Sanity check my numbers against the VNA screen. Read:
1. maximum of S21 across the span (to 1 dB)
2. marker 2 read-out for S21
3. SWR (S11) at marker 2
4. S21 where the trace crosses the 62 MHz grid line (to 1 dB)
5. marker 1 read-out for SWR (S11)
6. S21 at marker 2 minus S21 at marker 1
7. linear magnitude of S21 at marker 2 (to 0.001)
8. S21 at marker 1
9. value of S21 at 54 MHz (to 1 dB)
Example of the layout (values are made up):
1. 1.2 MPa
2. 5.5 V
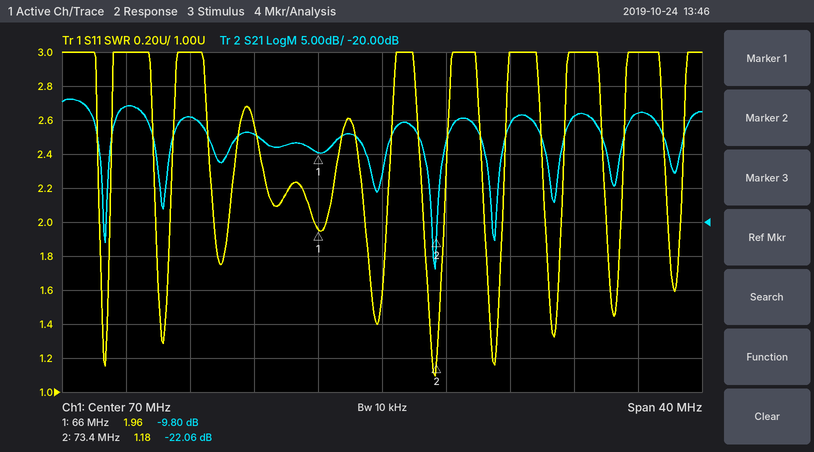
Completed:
1. -2 dB
2. -22.06 dB
3. 1.18
4. -7 dB
5. 1.96
6. -12.26 dB
7. 0.079
8. -9.80 dB
9. -3 dB
